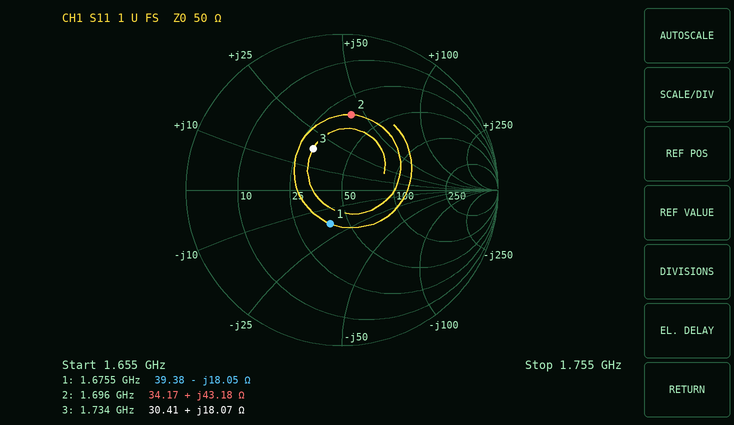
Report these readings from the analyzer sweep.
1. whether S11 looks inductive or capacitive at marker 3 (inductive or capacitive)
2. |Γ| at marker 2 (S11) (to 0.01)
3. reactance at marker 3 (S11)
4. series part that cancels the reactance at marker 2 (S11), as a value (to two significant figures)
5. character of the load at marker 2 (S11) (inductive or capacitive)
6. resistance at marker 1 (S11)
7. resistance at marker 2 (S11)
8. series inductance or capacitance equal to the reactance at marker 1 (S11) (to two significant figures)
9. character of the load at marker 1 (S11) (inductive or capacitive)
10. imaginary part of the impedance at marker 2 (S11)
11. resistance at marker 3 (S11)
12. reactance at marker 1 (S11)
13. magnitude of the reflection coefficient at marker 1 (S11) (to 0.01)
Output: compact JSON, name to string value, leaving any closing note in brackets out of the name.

{"whether S11 looks inductive or capacitive at marker 3": "inductive", "|Γ| at marker 2 (S11)": "0.49", "reactance at marker 3": "+18.07 Ω", "series part that cancels the reactance at marker 2 (S11), as a value": "2.2 pF", "character of the load at marker 2 (S11)": "inductive", "resistance at marker 1": "39.38 Ω", "resistance at marker 2": "34.17 Ω", "series inductance or capacitance equal to the reactance at marker 1 (S11)": "5.3 pF", "character of the load at marker 1 (S11)": "capacitive", "imaginary part of the impedance at marker 2": "+43.18 Ω", "resistance at marker 3": "30.41 Ω", "reactance at marker 1": "-18.05 Ω", "magnitude of the reflection coefficient at marker 1 (S11)": "0.23"}
